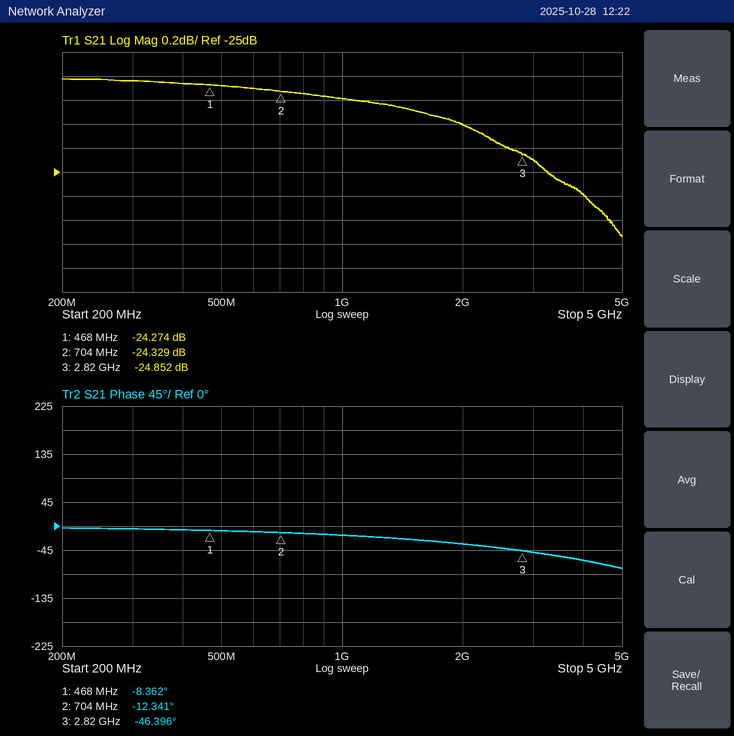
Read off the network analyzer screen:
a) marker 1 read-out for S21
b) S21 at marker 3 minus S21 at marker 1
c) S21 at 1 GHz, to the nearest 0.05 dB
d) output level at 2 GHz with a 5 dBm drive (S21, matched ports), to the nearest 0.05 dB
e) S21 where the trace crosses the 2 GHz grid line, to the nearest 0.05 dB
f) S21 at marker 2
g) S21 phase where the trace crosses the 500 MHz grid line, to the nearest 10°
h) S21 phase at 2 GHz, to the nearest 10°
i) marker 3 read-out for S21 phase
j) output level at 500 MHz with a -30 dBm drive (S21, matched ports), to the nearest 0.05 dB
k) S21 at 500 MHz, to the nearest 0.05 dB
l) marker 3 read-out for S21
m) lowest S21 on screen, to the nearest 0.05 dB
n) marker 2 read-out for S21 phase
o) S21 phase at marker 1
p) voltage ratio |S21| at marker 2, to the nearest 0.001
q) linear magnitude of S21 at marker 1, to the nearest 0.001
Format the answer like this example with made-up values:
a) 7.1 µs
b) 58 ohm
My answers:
a) -24.274 dB
b) -0.578 dB
c) -24.40 dB
d) -19.60 dBm
e) -24.60 dB
f) -24.329 dB
g) -10°
h) -30°
i) -46.396°
j) -54.30 dBm
k) -24.30 dB
l) -24.852 dB
m) -25.55 dB
n) -12.341°
o) -8.362°
p) 0.061
q) 0.061
